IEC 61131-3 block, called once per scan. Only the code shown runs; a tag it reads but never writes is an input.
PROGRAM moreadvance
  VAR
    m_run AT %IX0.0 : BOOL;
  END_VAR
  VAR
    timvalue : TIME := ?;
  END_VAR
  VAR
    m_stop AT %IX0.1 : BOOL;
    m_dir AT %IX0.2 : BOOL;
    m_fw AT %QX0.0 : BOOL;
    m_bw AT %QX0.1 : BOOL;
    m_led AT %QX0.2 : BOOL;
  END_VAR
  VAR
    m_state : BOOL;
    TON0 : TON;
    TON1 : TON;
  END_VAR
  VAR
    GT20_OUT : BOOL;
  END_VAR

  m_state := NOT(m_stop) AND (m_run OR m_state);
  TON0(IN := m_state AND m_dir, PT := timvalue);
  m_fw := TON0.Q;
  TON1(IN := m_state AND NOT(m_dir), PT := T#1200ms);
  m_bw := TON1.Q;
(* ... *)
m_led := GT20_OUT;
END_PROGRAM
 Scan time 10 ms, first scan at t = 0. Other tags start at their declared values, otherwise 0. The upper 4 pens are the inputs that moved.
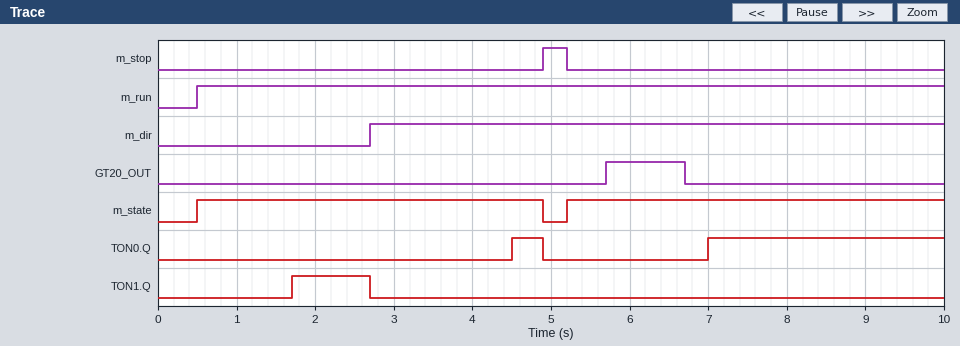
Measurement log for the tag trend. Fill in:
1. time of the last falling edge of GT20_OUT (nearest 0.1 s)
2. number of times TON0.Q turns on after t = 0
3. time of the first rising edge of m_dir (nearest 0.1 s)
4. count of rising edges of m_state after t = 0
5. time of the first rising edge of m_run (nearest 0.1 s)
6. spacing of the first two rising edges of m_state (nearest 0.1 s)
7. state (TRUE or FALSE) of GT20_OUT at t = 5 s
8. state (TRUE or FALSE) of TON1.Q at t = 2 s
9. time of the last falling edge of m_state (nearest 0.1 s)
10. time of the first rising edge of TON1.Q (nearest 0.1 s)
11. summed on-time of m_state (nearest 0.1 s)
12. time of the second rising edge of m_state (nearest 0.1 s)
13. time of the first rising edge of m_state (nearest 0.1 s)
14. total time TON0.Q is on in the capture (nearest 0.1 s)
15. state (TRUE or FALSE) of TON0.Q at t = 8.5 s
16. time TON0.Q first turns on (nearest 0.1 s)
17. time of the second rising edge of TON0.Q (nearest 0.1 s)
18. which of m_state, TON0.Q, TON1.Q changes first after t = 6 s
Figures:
6.7 s
2
2.7 s
2
0.5 s
4.7 s
FALSE
TRUE
4.9 s
1.7 s
9.2 s
5.2 s
0.5 s
3.4 s
TRUE
4.5 s
7.0 s
TON0.Q
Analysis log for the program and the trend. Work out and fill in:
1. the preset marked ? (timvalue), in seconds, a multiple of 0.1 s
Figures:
1.8 s
